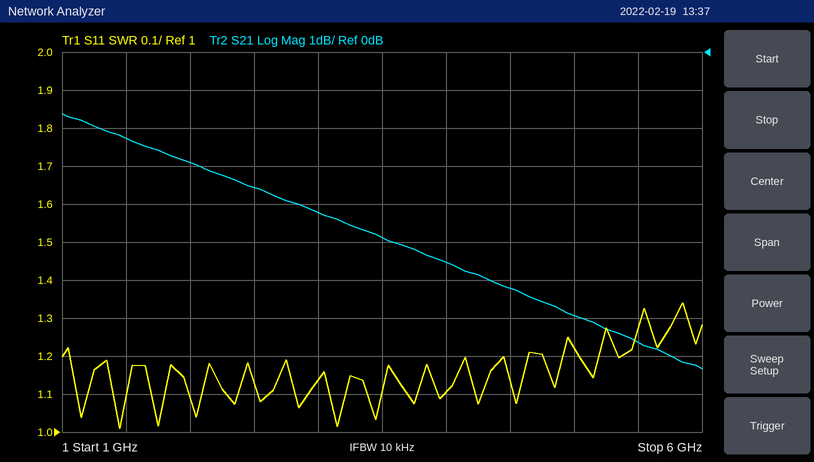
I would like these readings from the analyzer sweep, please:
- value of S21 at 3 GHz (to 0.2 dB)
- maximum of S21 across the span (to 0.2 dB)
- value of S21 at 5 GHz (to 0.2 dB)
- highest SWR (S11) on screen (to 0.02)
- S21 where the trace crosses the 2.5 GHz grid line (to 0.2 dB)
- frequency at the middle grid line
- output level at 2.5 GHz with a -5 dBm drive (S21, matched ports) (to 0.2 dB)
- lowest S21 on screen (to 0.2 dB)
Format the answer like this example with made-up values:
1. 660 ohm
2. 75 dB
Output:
1. -4.2 dB
2. -1.6 dB
3. -7.0 dB
4. 1.34
5. -3.6 dB
6. 3.5 GHz
7. -8.6 dBm
8. -8.4 dB
